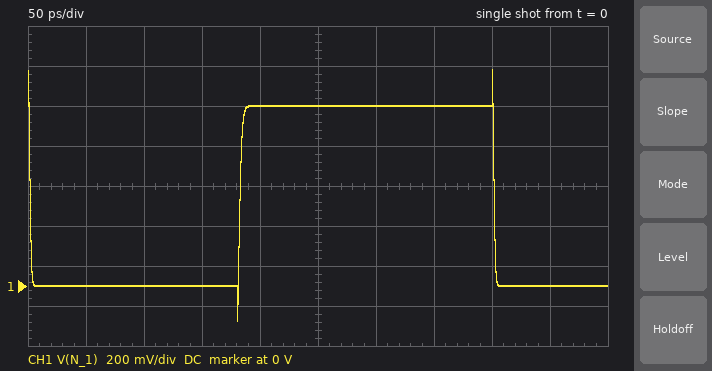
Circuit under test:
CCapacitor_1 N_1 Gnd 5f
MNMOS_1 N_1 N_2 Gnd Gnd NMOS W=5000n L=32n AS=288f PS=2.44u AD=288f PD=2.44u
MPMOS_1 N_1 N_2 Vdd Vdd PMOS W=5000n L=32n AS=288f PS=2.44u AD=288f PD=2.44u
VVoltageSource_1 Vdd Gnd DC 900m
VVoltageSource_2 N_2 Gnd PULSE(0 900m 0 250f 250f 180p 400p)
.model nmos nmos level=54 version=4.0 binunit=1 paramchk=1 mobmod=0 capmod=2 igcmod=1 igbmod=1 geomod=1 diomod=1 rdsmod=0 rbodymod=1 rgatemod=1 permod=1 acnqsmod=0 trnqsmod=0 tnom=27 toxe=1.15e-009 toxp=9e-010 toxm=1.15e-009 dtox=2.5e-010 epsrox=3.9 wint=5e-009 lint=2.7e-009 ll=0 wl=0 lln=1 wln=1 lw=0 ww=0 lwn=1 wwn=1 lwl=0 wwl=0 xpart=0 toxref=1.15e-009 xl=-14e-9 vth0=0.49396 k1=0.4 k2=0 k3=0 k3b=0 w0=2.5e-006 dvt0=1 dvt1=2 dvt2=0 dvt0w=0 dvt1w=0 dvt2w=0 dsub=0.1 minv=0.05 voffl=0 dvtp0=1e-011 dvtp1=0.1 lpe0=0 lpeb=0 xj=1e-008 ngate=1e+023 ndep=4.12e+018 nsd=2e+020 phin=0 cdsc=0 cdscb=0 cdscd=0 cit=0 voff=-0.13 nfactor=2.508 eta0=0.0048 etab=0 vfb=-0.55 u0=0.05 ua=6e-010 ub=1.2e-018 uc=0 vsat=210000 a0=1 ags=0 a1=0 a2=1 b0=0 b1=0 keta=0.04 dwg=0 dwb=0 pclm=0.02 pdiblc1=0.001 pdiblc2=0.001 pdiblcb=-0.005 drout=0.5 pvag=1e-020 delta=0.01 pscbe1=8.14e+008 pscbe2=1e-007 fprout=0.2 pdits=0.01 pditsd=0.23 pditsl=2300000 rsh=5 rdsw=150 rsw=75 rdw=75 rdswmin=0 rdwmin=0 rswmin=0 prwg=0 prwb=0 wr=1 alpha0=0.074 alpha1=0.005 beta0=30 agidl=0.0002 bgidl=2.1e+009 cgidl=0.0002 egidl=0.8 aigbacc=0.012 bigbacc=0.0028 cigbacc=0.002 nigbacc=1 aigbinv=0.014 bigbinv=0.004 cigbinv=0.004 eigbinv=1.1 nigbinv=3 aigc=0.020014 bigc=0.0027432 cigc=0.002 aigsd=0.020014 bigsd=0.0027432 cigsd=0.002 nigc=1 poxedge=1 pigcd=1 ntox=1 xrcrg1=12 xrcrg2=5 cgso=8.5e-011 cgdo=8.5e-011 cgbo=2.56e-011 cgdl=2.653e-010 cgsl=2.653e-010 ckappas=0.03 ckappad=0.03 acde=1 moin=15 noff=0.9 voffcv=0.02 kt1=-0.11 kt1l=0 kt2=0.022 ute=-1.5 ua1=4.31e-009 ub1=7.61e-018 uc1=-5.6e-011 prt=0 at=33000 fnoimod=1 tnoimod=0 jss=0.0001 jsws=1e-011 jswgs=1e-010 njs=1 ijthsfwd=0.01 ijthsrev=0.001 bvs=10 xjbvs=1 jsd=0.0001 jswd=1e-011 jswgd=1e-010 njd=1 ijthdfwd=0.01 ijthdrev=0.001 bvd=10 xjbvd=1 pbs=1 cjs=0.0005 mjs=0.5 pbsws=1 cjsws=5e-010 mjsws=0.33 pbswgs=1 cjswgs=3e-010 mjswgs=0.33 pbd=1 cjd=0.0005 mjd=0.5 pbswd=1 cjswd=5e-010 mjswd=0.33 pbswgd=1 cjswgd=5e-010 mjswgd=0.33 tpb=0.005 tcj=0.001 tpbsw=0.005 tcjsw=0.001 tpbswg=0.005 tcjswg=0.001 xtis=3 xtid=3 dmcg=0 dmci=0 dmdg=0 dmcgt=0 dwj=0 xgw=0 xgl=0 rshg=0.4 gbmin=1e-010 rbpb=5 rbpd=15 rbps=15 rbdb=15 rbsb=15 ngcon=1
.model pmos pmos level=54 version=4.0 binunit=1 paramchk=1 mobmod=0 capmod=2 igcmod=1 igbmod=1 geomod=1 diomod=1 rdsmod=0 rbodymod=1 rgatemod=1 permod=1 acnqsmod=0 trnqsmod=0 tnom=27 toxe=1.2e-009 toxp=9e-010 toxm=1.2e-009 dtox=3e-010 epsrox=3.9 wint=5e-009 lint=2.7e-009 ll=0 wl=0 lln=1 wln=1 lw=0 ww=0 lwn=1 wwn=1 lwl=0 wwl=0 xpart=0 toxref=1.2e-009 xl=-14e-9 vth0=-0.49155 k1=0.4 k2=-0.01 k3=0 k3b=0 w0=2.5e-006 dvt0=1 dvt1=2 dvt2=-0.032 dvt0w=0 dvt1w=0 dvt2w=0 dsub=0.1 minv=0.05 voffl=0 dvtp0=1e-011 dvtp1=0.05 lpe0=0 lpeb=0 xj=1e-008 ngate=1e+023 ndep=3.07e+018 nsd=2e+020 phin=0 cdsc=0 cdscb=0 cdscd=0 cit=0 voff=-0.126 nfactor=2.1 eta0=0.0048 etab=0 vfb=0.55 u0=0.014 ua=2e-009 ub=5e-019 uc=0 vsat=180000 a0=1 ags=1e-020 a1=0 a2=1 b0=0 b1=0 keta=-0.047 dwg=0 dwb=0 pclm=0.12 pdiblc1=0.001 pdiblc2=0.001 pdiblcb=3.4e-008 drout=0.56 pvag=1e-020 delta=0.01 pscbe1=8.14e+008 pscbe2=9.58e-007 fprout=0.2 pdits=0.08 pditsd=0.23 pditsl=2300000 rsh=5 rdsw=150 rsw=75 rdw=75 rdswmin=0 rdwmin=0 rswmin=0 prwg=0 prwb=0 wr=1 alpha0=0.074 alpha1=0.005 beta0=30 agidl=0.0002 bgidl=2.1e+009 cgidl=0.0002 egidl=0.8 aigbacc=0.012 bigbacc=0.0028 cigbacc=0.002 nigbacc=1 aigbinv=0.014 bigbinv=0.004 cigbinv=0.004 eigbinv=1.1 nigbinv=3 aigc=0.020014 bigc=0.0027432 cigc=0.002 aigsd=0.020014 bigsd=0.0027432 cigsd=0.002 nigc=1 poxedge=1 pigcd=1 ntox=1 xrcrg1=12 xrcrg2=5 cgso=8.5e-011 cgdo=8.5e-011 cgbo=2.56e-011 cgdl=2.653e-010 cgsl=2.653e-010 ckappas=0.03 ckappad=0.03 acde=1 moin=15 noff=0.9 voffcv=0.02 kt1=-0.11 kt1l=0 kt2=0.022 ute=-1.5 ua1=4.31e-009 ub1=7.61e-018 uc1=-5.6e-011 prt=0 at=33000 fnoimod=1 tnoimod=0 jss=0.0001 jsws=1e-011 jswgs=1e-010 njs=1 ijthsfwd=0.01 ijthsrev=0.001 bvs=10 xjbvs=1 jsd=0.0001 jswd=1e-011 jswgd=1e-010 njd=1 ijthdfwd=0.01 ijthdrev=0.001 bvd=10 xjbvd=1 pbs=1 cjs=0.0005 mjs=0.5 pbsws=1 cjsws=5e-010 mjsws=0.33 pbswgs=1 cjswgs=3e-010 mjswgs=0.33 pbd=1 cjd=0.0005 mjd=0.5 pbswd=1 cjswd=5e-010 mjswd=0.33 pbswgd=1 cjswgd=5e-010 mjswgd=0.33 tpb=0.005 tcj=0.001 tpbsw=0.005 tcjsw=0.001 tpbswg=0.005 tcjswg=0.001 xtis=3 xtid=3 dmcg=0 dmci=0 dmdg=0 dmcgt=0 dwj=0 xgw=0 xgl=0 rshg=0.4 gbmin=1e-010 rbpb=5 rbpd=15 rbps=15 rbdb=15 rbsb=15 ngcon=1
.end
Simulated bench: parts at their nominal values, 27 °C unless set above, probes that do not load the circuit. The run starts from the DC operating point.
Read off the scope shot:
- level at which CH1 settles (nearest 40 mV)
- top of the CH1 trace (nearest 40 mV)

0 V
1.08 V
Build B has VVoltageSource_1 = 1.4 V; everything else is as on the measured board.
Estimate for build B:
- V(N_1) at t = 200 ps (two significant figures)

1.4 V
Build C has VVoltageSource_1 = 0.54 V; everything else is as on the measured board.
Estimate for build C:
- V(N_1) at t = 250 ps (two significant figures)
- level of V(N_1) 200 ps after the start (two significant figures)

540 mV
460 mV
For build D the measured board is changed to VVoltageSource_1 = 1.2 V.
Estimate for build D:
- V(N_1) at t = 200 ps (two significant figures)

1.2 V
